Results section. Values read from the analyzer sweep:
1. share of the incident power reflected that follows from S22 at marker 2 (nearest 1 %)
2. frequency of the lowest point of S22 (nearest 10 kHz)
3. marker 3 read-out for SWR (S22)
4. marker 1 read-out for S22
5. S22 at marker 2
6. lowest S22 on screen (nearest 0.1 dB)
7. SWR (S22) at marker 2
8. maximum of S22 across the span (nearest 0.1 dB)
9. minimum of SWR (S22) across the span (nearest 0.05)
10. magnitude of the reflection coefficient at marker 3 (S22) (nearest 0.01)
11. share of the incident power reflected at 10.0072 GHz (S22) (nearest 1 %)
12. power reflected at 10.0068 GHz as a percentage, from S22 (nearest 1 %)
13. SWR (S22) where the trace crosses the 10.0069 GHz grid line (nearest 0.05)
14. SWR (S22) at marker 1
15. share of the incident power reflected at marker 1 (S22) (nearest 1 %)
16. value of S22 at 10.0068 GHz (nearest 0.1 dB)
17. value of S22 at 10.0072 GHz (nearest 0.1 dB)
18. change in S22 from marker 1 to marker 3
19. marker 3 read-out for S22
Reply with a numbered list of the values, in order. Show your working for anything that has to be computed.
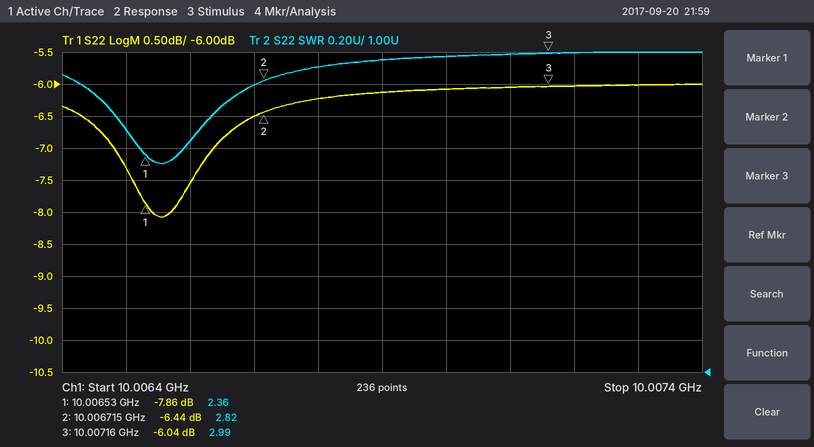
1. 10^(-6.44/10) ≈ 23 %
2. 10.00656 GHz
3. 2.99
4. -7.86 dB
5. -6.44 dB
6. -8.1 dB
7. 2.82
8. -6.0 dB
9. 2.30
10. 10^(-6.04/20) ≈ 0.50
11. 10^(-6/10) ≈ 25 %
12. 10^(-6.2/10) ≈ 24 %
13. 2.95
14. 2.36
15. 10^(-7.86/10) ≈ 16 %
16. -6.2 dB
17. -6.0 dB
18. -6.04 − (-7.86) = 1.82 dB
19. -6.04 dB
